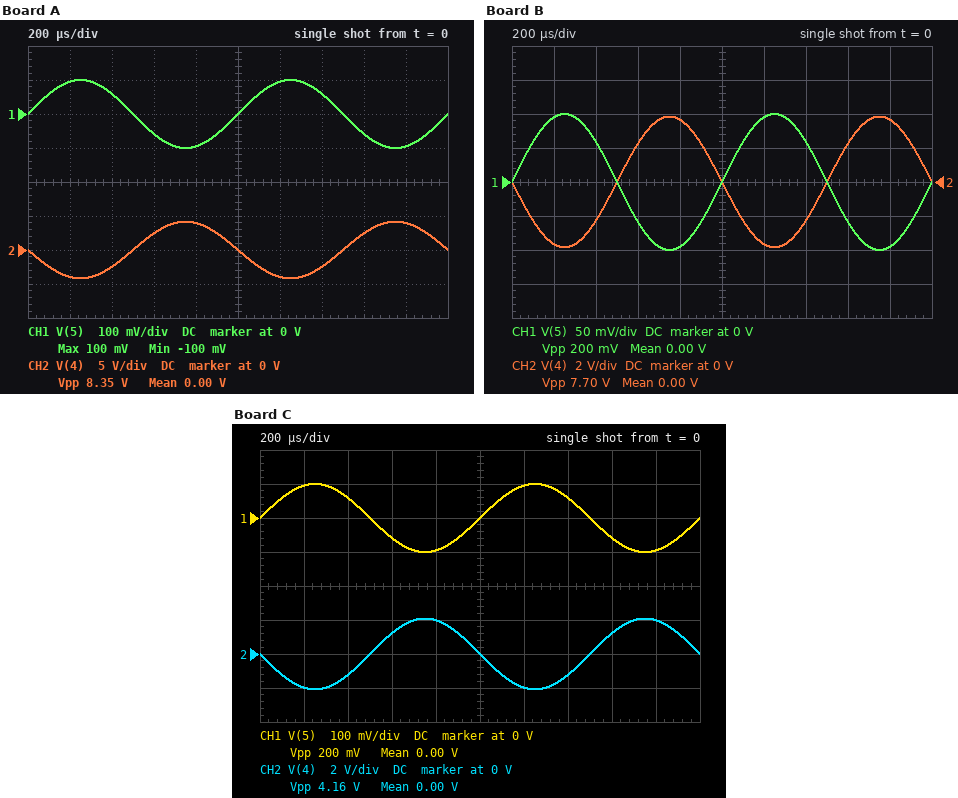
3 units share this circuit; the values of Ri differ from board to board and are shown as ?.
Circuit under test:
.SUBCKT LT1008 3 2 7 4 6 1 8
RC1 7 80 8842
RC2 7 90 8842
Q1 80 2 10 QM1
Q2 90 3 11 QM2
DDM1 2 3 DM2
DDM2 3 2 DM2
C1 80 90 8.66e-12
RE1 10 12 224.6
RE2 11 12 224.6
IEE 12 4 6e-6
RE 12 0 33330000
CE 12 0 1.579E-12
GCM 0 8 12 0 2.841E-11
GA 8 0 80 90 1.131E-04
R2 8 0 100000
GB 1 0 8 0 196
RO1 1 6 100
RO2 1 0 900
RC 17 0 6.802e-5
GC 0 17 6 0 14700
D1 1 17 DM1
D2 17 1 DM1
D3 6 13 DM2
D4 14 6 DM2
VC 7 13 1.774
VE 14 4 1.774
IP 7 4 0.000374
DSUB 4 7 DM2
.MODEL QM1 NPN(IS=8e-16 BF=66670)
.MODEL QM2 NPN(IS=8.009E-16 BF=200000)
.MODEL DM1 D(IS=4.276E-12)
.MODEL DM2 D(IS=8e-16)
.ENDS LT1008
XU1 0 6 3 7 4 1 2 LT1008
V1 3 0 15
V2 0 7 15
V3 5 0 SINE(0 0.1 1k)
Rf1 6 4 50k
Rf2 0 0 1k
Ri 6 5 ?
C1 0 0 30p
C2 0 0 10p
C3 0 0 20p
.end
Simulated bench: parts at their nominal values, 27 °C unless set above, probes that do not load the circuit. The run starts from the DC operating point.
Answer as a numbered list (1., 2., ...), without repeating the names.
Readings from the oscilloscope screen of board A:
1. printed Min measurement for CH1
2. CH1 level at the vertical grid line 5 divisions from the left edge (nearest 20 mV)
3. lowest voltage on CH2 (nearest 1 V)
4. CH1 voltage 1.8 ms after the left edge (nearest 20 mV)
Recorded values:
1. -100 mV
2. 0 V
3. -4 V
4. -100 mV
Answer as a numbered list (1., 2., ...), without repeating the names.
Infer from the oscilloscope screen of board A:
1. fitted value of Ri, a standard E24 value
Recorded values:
1. 1.2 kΩ
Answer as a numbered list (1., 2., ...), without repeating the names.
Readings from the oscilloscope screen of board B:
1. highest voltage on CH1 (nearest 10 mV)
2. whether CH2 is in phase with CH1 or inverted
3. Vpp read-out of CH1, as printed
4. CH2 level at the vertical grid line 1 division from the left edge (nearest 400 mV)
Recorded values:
1. 100 mV
2. inverted
3. 200 mV
4. -3.6 V
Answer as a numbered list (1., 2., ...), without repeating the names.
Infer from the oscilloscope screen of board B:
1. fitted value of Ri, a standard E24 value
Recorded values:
1. 1.3 kΩ
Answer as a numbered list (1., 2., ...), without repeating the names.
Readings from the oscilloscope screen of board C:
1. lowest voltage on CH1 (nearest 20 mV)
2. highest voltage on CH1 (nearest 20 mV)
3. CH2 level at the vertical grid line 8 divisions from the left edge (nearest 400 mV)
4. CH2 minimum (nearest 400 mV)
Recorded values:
1. -100 mV
2. 100 mV
3. 1.2 V
4. -2.0 V
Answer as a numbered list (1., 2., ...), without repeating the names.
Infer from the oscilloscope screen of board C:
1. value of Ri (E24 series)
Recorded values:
1. 2.4 kΩ
